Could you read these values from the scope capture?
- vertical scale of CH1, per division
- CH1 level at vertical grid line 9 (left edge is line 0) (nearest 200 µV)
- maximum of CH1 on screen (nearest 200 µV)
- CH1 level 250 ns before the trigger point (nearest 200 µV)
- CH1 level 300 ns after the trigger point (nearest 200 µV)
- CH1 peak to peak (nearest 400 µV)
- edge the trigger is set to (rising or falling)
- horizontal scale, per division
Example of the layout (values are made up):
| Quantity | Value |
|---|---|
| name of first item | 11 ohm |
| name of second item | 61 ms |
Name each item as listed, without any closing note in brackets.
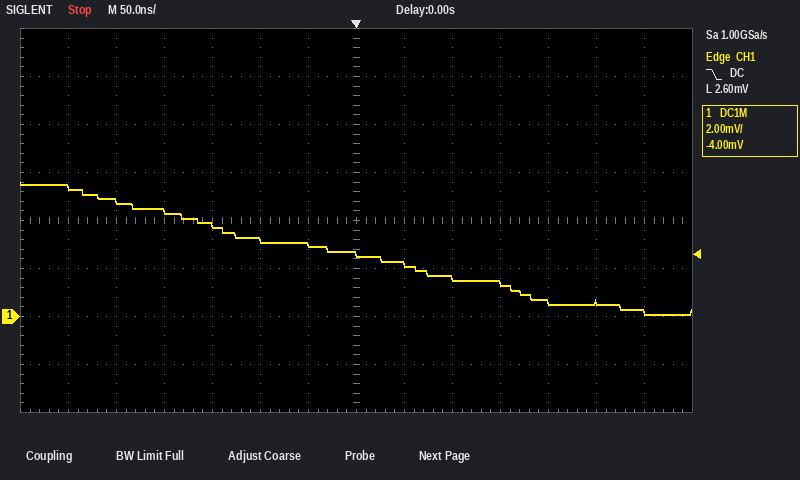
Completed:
| Quantity | Value |
|---|---|
| vertical scale of CH1, per division | 2 mV |
| CH1 level at vertical grid line 9 (left edge is line 0) | 1.6 mV |
| maximum of CH1 on screen | 5.6 mV |
| CH1 level 250 ns before the trigger point | 4.8 mV |
| CH1 level 300 ns after the trigger point | 200 µV |
| CH1 peak to peak | 5.6 mV |
| edge the trigger is set to | falling |
| horizontal scale, per division | 50 ns |
